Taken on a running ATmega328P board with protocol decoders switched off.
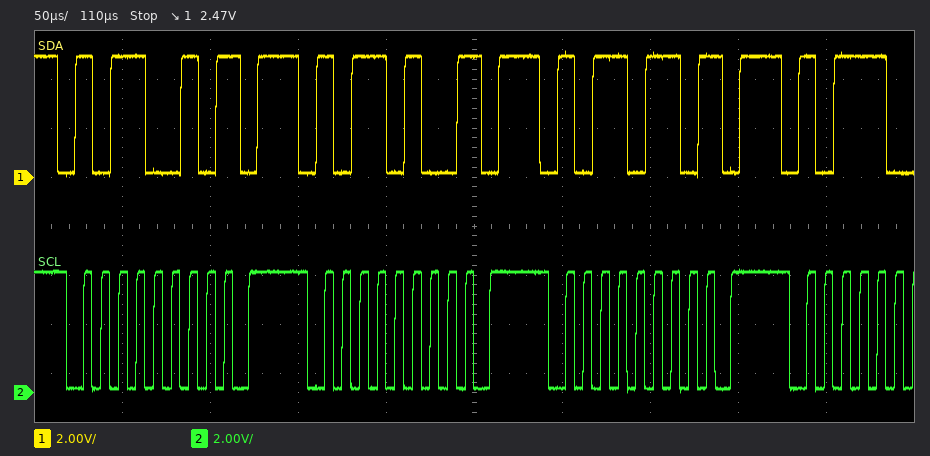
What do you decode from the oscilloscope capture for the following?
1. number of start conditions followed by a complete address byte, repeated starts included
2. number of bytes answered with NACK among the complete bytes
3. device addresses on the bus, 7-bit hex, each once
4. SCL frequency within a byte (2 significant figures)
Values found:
3
3
0x59 0x5A 0x5B
100 kHz
